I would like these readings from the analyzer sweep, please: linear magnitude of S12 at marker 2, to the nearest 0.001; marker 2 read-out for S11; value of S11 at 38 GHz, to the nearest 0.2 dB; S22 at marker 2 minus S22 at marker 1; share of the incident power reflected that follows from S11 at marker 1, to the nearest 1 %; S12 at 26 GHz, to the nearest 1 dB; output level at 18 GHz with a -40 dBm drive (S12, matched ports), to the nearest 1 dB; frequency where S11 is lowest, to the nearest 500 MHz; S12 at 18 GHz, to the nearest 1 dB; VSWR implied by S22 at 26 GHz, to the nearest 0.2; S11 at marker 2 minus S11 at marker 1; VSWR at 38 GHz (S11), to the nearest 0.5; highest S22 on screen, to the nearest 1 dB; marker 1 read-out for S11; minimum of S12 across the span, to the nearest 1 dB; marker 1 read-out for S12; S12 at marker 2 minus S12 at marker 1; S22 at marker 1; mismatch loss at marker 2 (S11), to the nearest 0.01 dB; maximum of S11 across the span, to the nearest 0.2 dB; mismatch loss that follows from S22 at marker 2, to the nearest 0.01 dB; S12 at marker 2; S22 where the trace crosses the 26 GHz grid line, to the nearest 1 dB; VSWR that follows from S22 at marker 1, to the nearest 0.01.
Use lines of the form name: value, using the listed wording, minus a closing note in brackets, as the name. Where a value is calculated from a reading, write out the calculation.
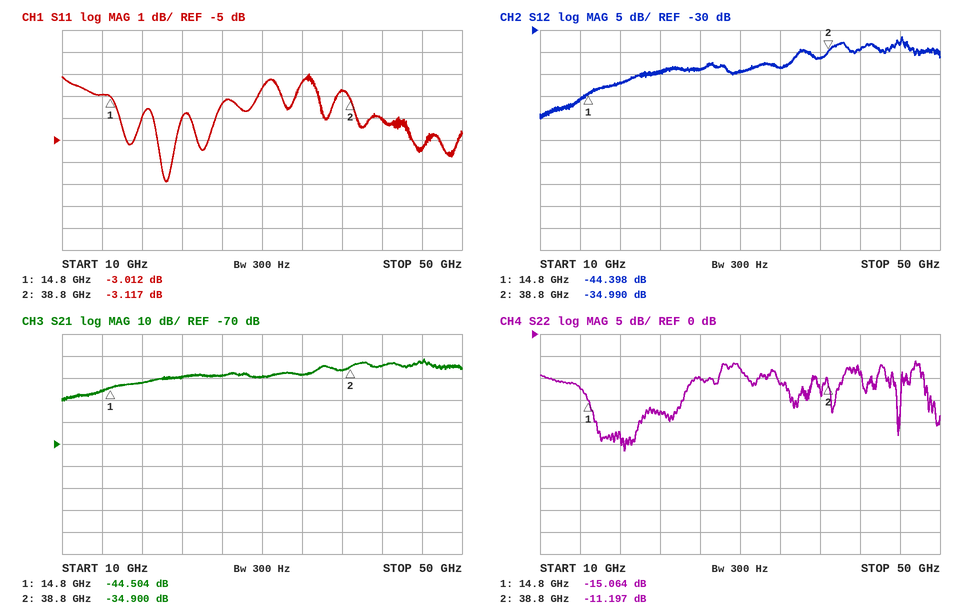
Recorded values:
linear magnitude of S12 at marker 2, to the nearest 0.001: 10^(-34.99/20) ≈ 0.018
marker 2 read-out for S11: -3.117 dB
value of S11 at 38 GHz, to the nearest 0.2 dB: -2.8 dB
S22 at marker 2 minus S22 at marker 1: -11.197 − (-15.064) = 3.867 dB
share of the incident power reflected that follows from S11 at marker 1, to the nearest 1 %: 10^(-3.012/10) ≈ 50 %
S12 at 26 GHz, to the nearest 1 dB: -39 dB
output level at 18 GHz with a -40 dBm drive (S12, matched ports), to the nearest 1 dB: -40 dBm + (-42 dB) = -82 dBm
frequency where S11 is lowest, to the nearest 500 MHz: 20.5 GHz
S12 at 18 GHz, to the nearest 1 dB: -42 dB
VSWR implied by S22 at 26 GHz, to the nearest 0.2: |Γ| = 10^(-10/20) = 0.3162; VSWR = (1 + 0.3162)/(1 − 0.3162) ≈ 1.92, so 2.0 to the nearest 0.2
S11 at marker 2 minus S11 at marker 1: -3.117 − (-3.012) = -0.105 dB
VSWR at 38 GHz (S11), to the nearest 0.5: |Γ| = 10^(-2.8/20) = 0.7244; VSWR = (1 + 0.7244)/(1 − 0.7244) ≈ 6.26, so 6.5 to the nearest 0.5
highest S22 on screen, to the nearest 1 dB: -6 dB
marker 1 read-out for S11: -3.012 dB
minimum of S12 across the span, to the nearest 1 dB: -50 dB
marker 1 read-out for S12: -44.398 dB
S12 at marker 2 minus S12 at marker 1: -34.99 − (-44.398) = 9.408 dB
S22 at marker 1: -15.064 dB
mismatch loss at marker 2 (S11), to the nearest 0.01 dB: −10 log10(1 − 10^(-3.117/10)) ≈ 2.91 dB
maximum of S11 across the span, to the nearest 0.2 dB: -2.0 dB
mismatch loss that follows from S22 at marker 2, to the nearest 0.01 dB: −10 log10(1 − 10^(-11.197/10)) ≈ 0.34 dB
S12 at marker 2: -34.990 dB
S22 where the trace crosses the 26 GHz grid line, to the nearest 1 dB: -10 dB
VSWR that follows from S22 at marker 1, to the nearest 0.01: (1 + 0.1765)/(1 − 0.1765) ≈ 1.43
